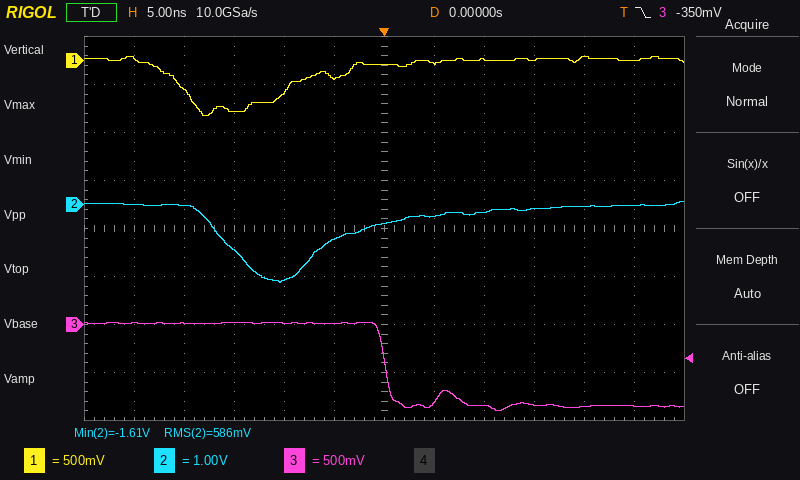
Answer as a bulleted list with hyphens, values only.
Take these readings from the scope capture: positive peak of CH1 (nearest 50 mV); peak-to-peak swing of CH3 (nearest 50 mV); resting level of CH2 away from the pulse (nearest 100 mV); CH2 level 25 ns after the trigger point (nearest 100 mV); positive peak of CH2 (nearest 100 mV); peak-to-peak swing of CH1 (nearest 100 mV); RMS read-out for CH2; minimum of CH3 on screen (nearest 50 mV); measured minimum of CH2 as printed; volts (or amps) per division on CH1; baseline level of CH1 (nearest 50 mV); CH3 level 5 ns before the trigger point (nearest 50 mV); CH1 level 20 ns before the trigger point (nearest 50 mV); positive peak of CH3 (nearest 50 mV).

- 50 mV
- 900 mV
- -100 mV
- 0.0 V
- 100 mV
- 600 mV
- 586 mV
- -900 mV
- -1.61 V
- 500 mV
- 0 mV
- 0 mV
- -300 mV
- 0 mV
